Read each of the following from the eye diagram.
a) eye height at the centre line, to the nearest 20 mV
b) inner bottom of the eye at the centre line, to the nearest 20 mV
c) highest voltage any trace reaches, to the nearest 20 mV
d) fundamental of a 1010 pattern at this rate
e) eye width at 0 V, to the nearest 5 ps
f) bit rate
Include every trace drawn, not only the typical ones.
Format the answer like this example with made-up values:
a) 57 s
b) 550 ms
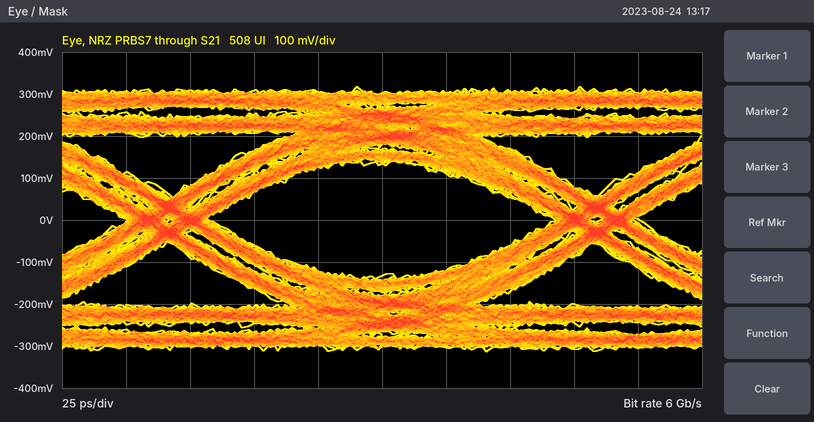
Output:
a) 260 mV
b) -140 mV
c) 320 mV
d) 3 GHz
e) 135 ps
f) 6 Gb/s
